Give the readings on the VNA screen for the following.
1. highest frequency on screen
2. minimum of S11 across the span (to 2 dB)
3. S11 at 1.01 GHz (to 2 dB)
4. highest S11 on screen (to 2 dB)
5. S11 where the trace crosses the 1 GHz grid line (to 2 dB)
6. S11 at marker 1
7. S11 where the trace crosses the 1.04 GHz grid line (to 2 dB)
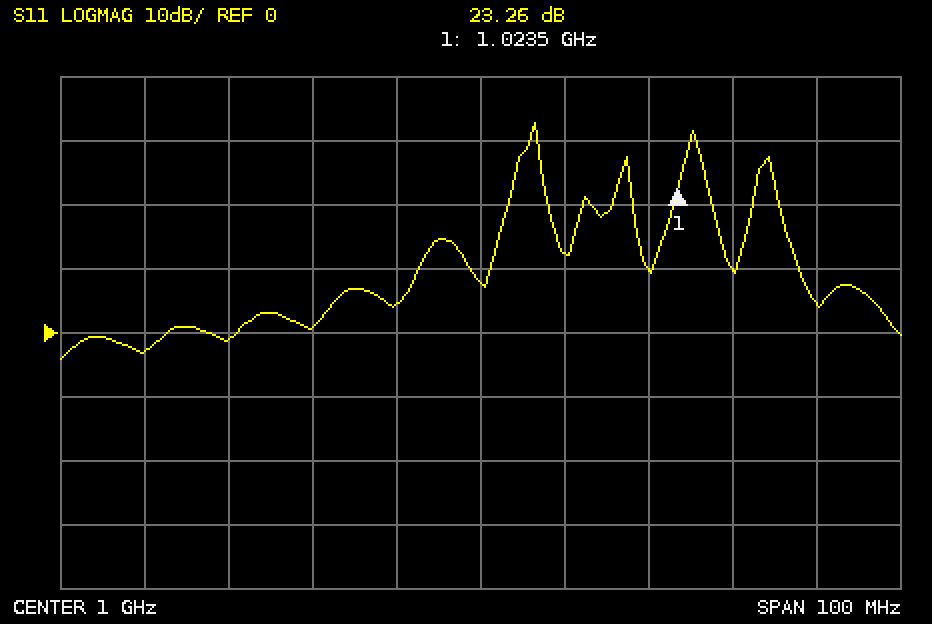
1.05 GHz
-4 dB
12 dB
32 dB
8 dB
23.26 dB
4 dB
